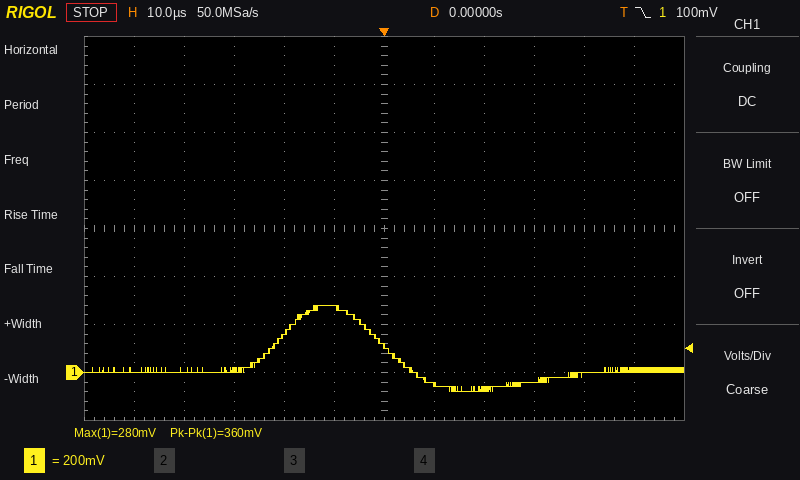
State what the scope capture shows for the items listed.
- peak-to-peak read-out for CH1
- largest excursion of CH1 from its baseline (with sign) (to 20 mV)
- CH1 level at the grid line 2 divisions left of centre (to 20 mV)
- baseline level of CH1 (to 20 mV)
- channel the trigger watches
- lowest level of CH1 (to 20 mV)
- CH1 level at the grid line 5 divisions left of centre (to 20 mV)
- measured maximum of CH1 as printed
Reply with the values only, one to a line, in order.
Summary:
360 mV
+280 mV
160 mV
0 mV
CH1
-80 mV
0 mV
280 mV
